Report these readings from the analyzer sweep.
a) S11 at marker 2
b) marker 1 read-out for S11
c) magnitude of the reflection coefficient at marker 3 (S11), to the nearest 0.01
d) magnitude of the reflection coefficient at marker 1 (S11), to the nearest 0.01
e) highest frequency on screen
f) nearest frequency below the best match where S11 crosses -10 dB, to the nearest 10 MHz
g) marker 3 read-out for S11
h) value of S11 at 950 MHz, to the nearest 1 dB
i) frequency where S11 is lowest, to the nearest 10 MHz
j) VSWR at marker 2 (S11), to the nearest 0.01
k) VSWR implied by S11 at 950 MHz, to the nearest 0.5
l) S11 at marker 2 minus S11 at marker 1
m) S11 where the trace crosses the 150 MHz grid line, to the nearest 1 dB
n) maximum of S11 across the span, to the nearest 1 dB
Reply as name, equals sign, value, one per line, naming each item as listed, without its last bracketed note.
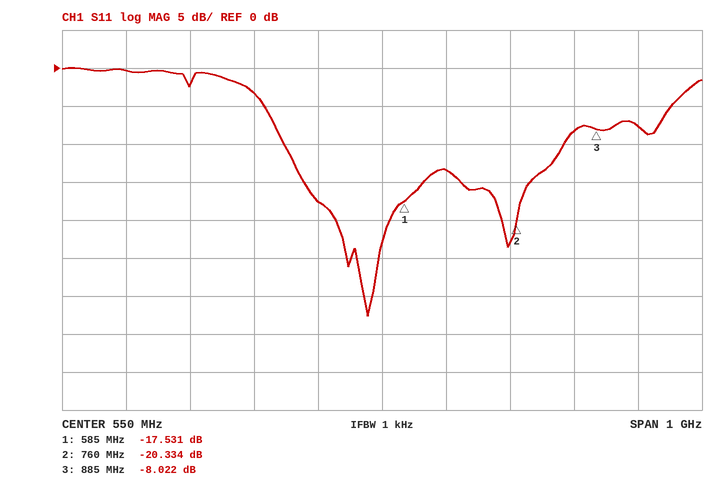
S11 at marker 2 = -20.334 dB
marker 1 read-out for S11 = -17.531 dB
magnitude of the reflection coefficient at marker 3 (S11), to the nearest 0.01 = 0.40
magnitude of the reflection coefficient at marker 1 (S11), to the nearest 0.01 = 0.13
highest frequency on screen = 1.05 GHz
nearest frequency below the best match where S11 crosses -10 dB, to the nearest 10 MHz = 400 MHz
marker 3 read-out for S11 = -8.022 dB
value of S11 at 950 MHz, to the nearest 1 dB = -8 dB
frequency where S11 is lowest, to the nearest 10 MHz = 530 MHz
VSWR at marker 2 (S11), to the nearest 0.01 = 1.21
VSWR implied by S11 at 950 MHz, to the nearest 0.5 = 2.5
S11 at marker 2 minus S11 at marker 1 = -2.803 dB
S11 where the trace crosses the 150 MHz grid line, to the nearest 1 dB = 0 dB
maximum of S11 across the span, to the nearest 1 dB = 0 dB
